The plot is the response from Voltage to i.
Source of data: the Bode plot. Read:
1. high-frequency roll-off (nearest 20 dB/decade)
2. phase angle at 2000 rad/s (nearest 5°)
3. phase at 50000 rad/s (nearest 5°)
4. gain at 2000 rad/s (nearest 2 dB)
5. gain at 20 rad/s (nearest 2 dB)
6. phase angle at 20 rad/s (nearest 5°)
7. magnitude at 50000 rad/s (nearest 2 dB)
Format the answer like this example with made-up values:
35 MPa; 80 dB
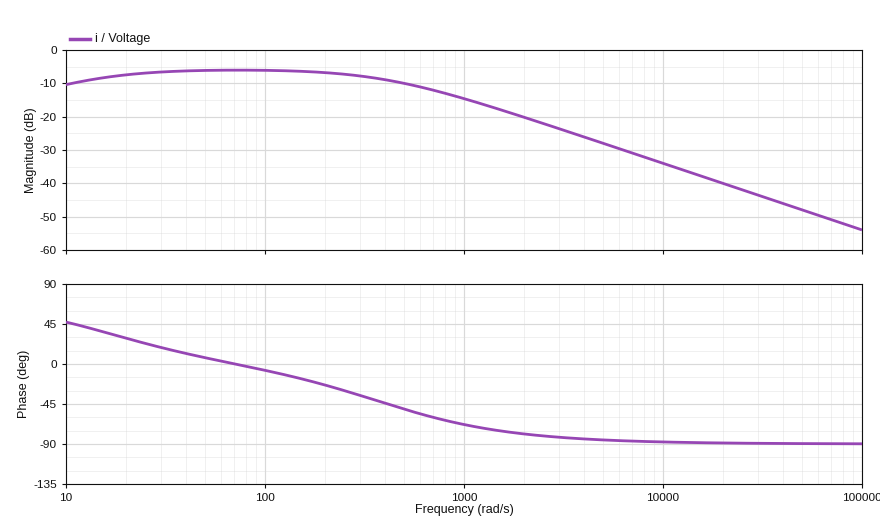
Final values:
-20 dB/decade; -80°; -90°; -20 dB; -8 dB; 30°; -48 dB
